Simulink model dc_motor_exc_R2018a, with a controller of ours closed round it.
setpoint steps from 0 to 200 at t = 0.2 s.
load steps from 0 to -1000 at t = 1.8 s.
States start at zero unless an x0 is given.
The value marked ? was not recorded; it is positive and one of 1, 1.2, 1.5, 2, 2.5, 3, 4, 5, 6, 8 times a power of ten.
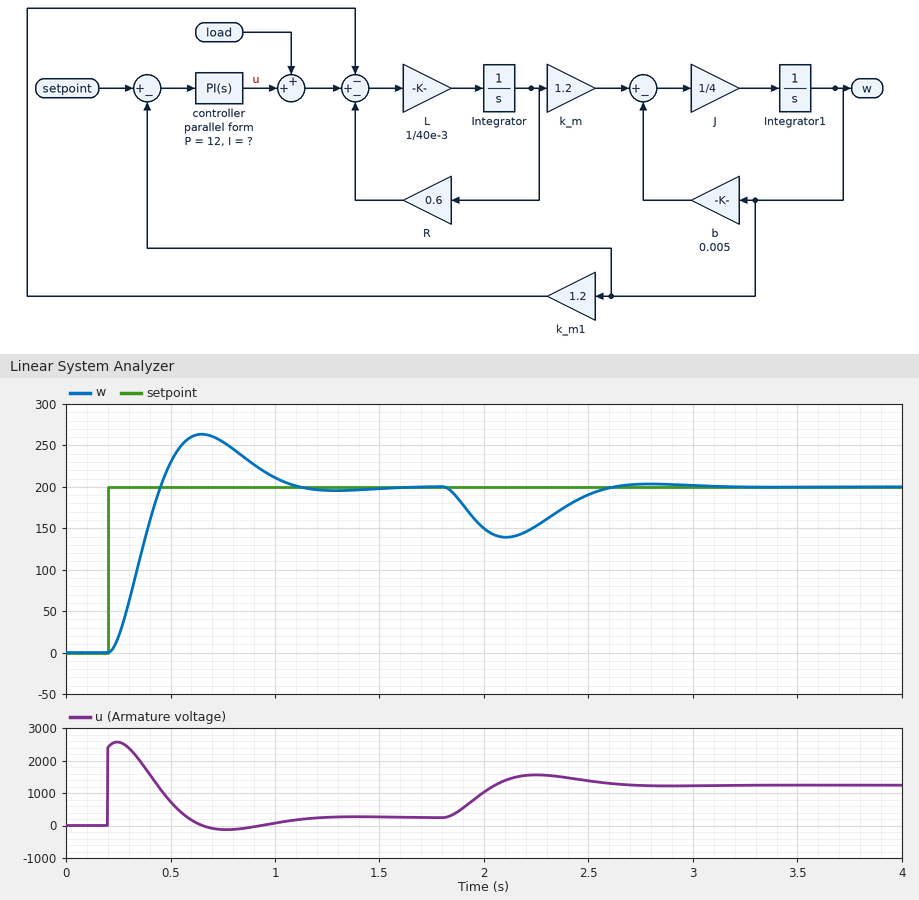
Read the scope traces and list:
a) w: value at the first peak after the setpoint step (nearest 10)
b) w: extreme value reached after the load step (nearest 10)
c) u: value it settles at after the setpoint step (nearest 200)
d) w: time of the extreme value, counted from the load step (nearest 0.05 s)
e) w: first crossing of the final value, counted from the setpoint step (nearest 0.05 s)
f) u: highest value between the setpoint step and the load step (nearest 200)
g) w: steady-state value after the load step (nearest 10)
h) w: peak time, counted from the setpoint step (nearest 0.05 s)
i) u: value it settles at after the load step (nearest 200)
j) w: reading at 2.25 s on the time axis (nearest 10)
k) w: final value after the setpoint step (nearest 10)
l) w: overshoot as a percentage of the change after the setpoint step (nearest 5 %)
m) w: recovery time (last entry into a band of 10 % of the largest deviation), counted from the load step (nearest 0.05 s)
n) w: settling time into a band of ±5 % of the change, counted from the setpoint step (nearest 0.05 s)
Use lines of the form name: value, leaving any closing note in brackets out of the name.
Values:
w: value at the first peak after the setpoint step: 260
w: extreme value reached after the load step: 140
u: value it settles at after the setpoint step: 200
w: time of the extreme value, counted from the load step: 0.30 s
w: first crossing of the final value, counted from the setpoint step: 0.25 s
u: highest value between the setpoint step and the load step: 2600
w: steady-state value after the load step: 200
w: peak time, counted from the setpoint step: 0.45 s
u: value it settles at after the load step: 1200
w: reading at 2.25 s on the time axis: 150
w: final value after the setpoint step: 200
w: overshoot as a percentage of the change after the setpoint step: 30 %
w: recovery time (last entry into a band of 10 % of the largest deviation), counted from the load step: 0.75 s
w: settling time into a band of ±5 % of the change, counted from the setpoint step: 0.80 s
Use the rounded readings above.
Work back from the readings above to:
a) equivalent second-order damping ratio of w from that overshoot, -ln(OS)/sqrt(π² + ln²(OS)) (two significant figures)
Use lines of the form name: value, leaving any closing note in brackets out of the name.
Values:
equivalent second-order damping ratio of w from that overshoot, -ln(OS)/sqrt(π² + ln²(OS)): 0.36
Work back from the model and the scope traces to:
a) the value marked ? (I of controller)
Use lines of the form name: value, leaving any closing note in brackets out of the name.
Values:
the value marked ?: 40
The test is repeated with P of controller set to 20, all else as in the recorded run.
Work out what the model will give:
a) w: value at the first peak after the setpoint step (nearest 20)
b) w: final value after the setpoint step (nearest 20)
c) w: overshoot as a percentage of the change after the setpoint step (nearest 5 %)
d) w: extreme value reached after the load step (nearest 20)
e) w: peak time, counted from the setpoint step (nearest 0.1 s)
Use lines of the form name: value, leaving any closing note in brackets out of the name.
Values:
w: value at the first peak after the setpoint step: 240
w: final value after the setpoint step: 200
w: overshoot as a percentage of the change after the setpoint step: 25 %
w: extreme value reached after the load step: 160
w: peak time, counted from the setpoint step: 0.3 s
